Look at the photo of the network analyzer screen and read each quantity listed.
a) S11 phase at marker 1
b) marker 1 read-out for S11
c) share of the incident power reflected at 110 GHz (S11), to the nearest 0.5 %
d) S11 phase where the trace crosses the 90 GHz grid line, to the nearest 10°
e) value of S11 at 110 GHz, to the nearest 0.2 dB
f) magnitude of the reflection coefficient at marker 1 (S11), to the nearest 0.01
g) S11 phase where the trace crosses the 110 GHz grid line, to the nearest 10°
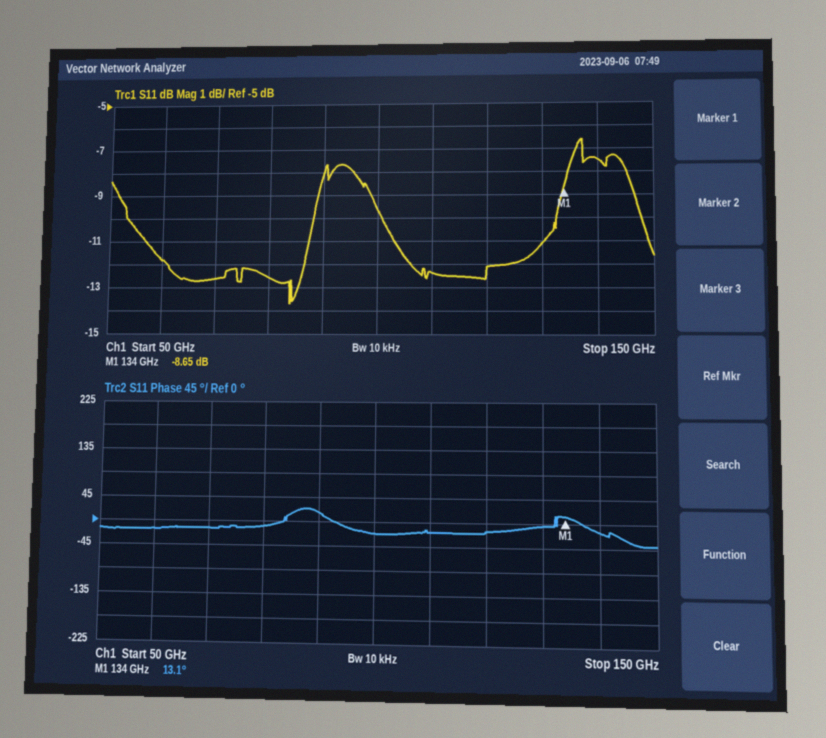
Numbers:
13.1°
-8.65 dB
6.0 %
20°
-12.4 dB
0.37
-20°
